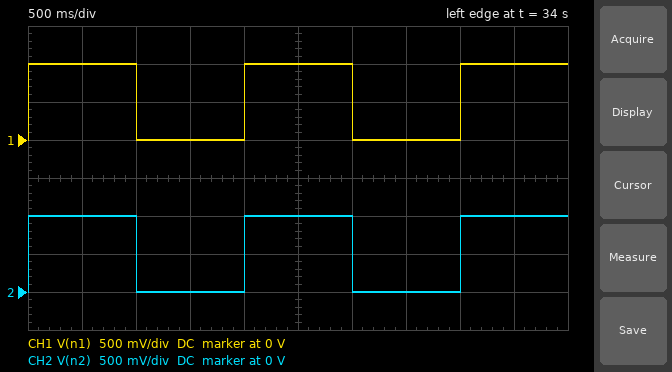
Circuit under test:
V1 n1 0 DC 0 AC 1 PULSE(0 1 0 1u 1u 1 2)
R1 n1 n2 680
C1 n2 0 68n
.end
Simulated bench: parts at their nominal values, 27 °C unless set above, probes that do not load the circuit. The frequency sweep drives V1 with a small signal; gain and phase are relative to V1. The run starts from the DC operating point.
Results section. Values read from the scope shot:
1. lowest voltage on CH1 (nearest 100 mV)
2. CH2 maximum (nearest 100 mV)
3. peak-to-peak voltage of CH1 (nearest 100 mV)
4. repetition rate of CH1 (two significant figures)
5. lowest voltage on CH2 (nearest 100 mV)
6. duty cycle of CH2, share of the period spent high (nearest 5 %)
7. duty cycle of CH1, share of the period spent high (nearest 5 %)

0 V
1.0 V
1.0 V
500 mHz
0 V
50 %
50 %
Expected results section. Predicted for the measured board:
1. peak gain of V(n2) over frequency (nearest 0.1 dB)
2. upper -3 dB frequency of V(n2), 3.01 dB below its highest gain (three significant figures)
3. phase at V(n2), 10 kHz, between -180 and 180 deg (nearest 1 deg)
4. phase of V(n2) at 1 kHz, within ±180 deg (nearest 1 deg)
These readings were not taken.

0 dB
3.44 kHz
-71 deg
-16 deg
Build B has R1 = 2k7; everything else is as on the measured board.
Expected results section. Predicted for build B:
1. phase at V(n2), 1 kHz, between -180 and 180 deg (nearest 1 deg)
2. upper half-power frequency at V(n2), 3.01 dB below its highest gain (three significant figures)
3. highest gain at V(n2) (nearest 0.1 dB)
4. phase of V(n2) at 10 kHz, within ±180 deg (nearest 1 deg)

-49 deg
867 Hz
0 dB
-85 deg
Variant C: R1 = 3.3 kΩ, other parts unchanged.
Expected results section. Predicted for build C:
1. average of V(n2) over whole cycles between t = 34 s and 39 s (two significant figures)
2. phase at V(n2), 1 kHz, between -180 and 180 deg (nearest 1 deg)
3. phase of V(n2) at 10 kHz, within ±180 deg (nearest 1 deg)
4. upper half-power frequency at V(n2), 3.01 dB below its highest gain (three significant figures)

500 mV
-55 deg
-86 deg
709 Hz
